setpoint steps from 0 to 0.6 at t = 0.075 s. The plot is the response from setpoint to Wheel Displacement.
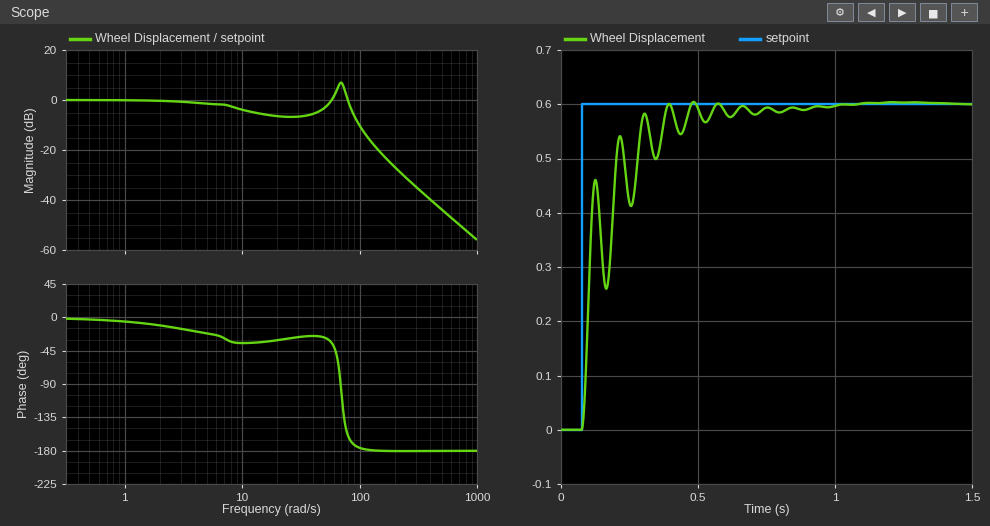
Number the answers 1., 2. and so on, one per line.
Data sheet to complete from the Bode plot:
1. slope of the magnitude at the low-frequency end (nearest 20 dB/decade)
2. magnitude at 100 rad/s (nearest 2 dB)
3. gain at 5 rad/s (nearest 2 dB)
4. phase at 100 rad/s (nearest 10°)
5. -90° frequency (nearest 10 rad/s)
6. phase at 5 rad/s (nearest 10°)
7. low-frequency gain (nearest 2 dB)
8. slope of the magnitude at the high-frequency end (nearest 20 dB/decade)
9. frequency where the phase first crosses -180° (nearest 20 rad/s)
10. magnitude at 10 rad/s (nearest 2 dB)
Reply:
1. 0 dB/decade
2. -10 dB
3. -2 dB
4. -180°
5. 70 rad/s
6. -20°
7. 0 dB
8. -40 dB/decade
9. 140 rad/s
10. -4 dB
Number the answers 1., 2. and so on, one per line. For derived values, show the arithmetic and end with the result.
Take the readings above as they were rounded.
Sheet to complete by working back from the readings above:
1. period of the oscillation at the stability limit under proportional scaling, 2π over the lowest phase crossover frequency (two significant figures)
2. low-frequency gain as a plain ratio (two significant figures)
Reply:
1. 2π / 140 = 0.045 s
2. 10^(0 / 20) = 1.0
